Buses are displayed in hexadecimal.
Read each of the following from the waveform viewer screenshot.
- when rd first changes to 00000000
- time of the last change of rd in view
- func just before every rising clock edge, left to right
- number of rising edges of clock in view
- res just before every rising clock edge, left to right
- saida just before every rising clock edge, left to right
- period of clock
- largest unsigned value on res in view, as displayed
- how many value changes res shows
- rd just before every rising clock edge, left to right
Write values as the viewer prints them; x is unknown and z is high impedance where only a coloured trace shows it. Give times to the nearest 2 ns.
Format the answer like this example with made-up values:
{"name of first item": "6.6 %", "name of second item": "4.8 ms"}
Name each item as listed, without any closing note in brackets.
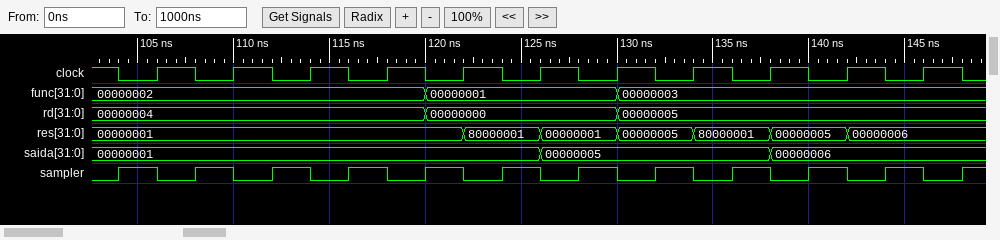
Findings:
{"when rd first changes to 00000000": "120 ns", "time of the last change of rd in view": "130 ns", "func just before every rising clock edge, left to right": "00000002, 00000002, 00000002, 00000002, 00000001, 00000001, 00000001, 00000003, 00000003, 00000003, 00000003", "number of rising edges of clock in view": "11", "res just before every rising clock edge, left to right": "00000001, 00000001, 00000001, 00000001, 00000001, 80000001, 00000001, 00000005, 80000001, 00000005, 00000006", "saida just before every rising clock edge, left to right": "00000001, 00000001, 00000001, 00000001, 00000001, 00000001, 00000005, 00000005, 00000005, 00000006, 00000006", "period of clock": "4 ns", "largest unsigned value on res in view, as displayed": "80000001", "how many value changes res shows": "6", "rd just before every rising clock edge, left to right": "00000004, 00000004, 00000004, 00000004, 00000000, 00000000, 00000000, 00000005, 00000005, 00000005, 00000005"}
